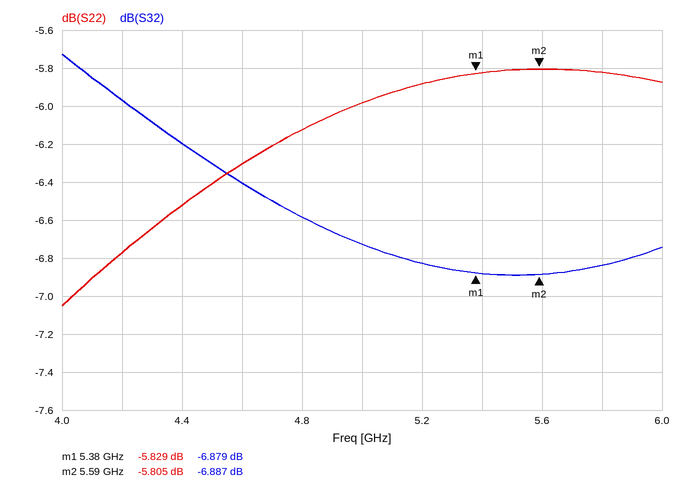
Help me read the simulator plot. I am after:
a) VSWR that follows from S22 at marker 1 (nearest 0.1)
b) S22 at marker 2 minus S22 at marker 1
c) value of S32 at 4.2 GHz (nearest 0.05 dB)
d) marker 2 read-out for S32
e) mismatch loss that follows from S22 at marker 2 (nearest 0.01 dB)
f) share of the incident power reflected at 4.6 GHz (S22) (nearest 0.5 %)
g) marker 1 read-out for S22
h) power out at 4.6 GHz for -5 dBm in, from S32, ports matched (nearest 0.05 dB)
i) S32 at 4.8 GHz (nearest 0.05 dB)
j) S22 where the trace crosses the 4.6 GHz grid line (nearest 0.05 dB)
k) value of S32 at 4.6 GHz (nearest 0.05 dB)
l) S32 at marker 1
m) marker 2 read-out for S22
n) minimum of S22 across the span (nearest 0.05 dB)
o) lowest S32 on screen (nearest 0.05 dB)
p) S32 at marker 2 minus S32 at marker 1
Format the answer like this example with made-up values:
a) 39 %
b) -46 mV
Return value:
a) 3.1
b) 0.024 dB
c) -5.95 dB
d) -6.887 dB
e) 1.32 dB
f) 23.5 %
g) -5.829 dB
h) -11.40 dBm
i) -6.60 dB
j) -6.30 dB
k) -6.40 dB
l) -6.879 dB
m) -5.805 dB
n) -7.05 dB
o) -6.90 dB
p) -0.008 dB
